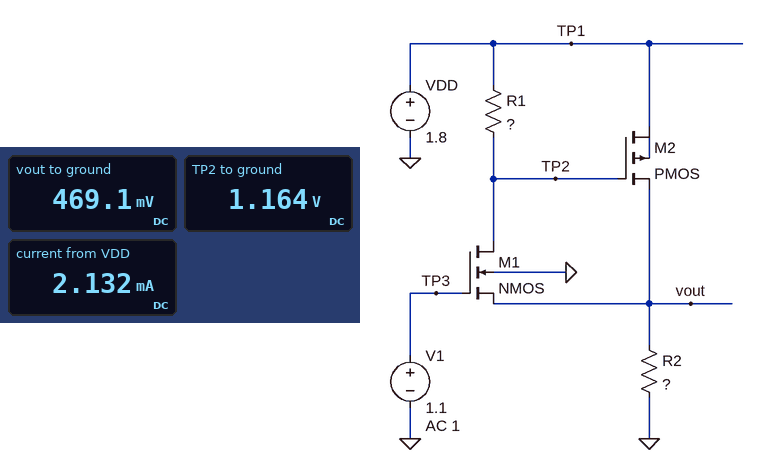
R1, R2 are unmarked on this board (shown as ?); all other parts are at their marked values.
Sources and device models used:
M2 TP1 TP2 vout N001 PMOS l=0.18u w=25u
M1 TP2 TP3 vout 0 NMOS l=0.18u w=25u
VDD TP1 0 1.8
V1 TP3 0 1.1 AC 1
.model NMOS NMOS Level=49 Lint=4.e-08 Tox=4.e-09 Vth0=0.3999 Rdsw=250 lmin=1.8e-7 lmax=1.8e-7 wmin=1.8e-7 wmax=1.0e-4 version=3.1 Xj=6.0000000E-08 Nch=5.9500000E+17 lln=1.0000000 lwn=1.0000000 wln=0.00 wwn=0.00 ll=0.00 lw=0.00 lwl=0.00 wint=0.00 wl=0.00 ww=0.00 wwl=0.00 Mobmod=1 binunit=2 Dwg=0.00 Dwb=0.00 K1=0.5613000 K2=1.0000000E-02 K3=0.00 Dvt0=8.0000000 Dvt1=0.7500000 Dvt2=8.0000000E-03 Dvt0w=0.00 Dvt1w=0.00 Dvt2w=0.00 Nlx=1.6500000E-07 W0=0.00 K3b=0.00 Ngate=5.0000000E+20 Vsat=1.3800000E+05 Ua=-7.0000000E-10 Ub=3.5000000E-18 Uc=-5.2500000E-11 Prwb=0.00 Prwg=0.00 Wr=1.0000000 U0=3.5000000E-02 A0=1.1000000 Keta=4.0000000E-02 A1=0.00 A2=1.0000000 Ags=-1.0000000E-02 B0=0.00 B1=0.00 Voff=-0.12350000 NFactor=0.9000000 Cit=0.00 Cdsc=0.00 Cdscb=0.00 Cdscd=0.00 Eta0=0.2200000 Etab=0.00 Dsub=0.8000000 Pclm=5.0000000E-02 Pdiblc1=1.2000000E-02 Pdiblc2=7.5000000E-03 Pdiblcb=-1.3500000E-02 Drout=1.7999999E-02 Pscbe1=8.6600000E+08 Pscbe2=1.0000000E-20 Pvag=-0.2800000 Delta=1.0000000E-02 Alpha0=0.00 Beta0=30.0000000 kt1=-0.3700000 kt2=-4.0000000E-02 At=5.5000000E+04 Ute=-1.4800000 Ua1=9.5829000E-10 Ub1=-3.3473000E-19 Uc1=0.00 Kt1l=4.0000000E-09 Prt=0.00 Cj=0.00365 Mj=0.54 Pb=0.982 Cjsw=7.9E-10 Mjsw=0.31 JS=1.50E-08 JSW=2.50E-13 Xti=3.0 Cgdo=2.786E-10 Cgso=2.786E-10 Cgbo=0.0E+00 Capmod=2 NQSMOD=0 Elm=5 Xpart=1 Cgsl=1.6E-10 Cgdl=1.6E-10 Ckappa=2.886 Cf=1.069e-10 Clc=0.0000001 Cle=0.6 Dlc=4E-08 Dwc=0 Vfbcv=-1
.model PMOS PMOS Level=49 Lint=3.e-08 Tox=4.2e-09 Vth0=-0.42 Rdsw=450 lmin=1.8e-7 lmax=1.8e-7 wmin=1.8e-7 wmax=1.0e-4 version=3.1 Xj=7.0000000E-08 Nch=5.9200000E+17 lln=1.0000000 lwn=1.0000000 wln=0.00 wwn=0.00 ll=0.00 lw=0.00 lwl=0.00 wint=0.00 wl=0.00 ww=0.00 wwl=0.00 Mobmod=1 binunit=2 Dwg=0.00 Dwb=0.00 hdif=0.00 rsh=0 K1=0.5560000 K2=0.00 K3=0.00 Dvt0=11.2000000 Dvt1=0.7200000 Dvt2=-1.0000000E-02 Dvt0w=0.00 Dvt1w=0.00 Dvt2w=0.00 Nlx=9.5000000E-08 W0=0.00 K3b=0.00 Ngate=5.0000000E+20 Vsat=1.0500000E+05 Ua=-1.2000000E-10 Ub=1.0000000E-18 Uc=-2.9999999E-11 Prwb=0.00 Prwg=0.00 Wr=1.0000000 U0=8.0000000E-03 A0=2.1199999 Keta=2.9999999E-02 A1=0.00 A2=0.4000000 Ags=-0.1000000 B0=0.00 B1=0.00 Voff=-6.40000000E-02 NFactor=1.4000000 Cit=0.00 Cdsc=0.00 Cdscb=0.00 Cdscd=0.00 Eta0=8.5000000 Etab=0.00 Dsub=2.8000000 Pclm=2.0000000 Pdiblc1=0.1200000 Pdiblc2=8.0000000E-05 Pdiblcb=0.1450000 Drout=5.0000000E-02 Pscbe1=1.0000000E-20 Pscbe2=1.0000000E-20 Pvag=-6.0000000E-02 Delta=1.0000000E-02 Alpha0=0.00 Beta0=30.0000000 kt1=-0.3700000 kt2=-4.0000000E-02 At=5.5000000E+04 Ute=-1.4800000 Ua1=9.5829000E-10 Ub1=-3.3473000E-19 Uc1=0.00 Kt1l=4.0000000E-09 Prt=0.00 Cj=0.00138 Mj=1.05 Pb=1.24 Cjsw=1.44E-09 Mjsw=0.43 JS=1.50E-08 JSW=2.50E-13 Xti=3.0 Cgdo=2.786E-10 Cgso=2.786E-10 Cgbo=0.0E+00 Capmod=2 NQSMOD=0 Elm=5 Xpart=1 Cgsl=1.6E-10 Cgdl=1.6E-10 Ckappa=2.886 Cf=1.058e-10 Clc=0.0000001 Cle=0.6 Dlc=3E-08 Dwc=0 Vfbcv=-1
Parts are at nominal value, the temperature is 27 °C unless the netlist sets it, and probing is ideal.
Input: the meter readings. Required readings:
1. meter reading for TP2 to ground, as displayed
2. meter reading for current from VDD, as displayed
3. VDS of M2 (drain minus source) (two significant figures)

1.164 V
2.132 mA
1.3 V
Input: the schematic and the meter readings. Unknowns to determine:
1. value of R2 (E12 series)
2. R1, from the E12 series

220 Ω
680 Ω
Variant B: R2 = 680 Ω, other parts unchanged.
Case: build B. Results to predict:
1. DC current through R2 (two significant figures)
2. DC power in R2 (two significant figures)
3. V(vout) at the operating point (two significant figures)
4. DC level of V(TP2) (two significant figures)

780 µA
410 µW
530 mV
1.4 V
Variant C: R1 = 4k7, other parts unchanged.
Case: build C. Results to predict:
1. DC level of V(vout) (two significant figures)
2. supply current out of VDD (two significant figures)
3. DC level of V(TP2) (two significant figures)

560 mV
2.6 mA
920 mV
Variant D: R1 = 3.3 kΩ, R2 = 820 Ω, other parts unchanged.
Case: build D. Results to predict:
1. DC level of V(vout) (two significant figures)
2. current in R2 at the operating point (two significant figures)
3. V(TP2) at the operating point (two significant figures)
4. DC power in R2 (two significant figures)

600 mV
730 µA
1.3 V
440 µW
